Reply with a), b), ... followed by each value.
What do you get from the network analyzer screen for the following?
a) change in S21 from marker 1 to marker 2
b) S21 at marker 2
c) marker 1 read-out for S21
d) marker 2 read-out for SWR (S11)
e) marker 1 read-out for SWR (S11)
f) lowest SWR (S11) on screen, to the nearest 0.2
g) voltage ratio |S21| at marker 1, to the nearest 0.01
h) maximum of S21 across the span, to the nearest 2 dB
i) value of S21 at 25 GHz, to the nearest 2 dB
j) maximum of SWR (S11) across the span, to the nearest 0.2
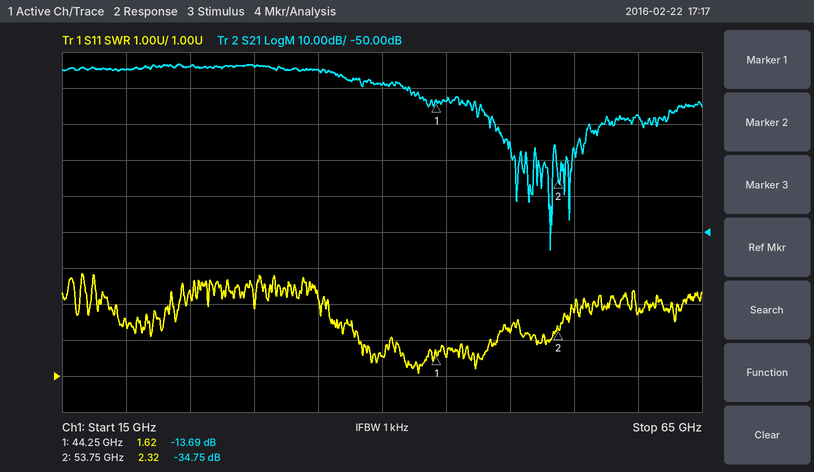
a) -21.06 dB
b) -34.75 dB
c) -13.69 dB
d) 2.32
e) 1.62
f) 1.0
g) 0.21
h) -4 dB
i) -4 dB
j) 3.8
